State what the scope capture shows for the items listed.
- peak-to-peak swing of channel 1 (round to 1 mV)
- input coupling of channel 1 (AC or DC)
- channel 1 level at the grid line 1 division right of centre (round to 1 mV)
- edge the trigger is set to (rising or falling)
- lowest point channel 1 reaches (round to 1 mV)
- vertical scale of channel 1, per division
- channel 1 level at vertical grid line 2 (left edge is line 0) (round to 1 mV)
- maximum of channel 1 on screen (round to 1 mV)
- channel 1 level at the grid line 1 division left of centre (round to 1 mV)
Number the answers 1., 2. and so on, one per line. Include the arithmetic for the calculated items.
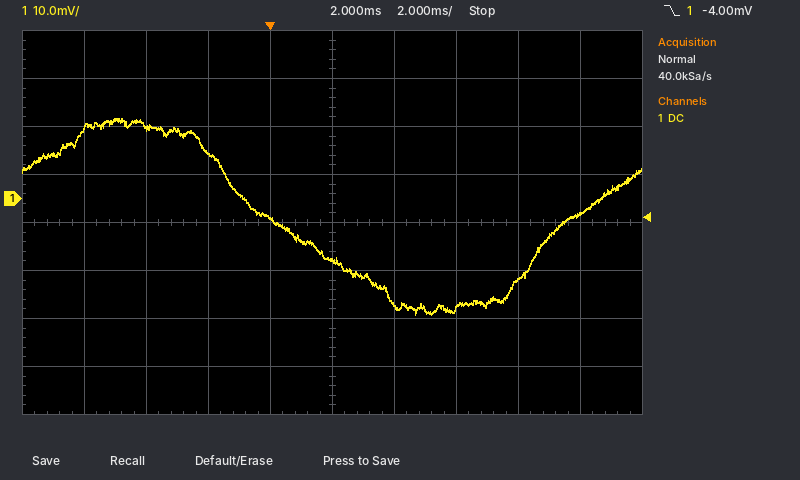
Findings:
1. 17 mV − (-24 mV) = 41 mV
2. DC
3. -22 mV
4. falling
5. -24 mV
6. 10 mV
7. 15 mV
8. 17 mV
9. -4 mV
